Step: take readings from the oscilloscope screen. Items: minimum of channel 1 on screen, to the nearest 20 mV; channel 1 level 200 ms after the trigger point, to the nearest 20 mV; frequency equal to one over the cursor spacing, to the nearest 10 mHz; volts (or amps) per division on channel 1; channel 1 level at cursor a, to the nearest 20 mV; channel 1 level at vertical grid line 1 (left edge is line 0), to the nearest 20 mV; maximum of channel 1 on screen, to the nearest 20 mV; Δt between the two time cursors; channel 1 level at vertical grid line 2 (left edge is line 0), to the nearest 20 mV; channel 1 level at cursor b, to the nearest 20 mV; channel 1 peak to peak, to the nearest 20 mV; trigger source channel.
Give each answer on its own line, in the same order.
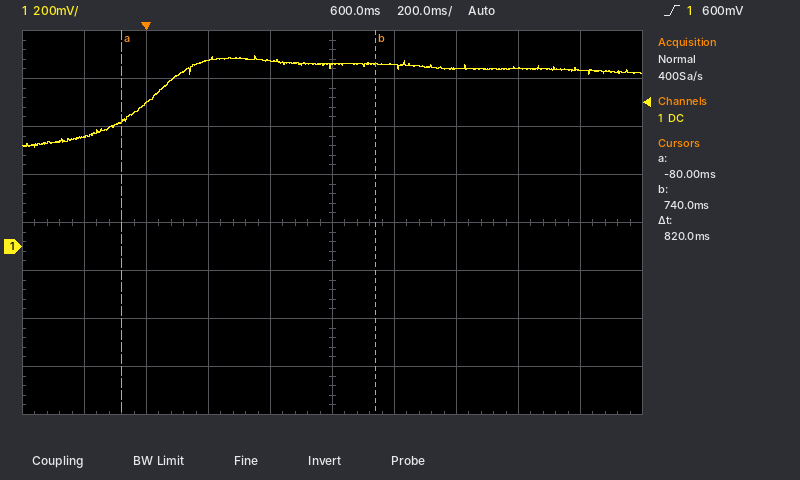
420 mV
780 mV
1.22 Hz
200 mV
520 mV
460 mV
800 mV
820 ms
600 mV
760 mV
380 mV
channel 1
